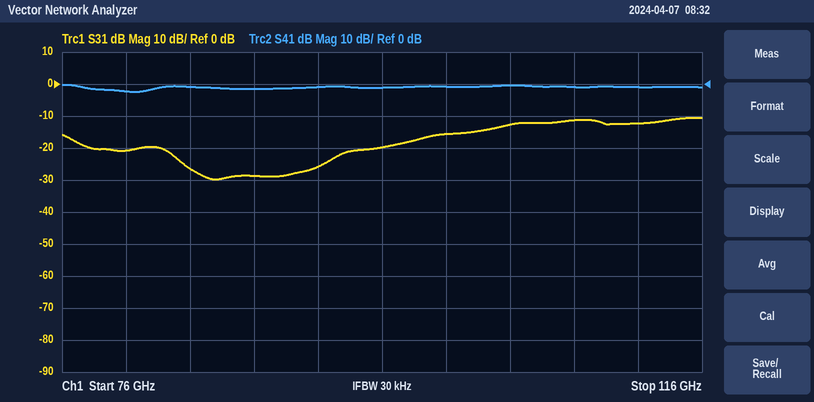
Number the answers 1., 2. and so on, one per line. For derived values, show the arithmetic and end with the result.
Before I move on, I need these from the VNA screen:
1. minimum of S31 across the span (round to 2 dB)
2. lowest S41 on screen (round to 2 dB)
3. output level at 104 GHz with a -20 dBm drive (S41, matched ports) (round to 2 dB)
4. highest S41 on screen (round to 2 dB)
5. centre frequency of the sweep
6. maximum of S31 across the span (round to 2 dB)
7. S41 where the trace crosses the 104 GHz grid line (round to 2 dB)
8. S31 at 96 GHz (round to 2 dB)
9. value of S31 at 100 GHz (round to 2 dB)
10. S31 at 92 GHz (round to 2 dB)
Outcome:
1. -30 dB
2. -2 dB
3. -20 dBm + (0 dB) = -20 dBm
4. 0 dB
5. 96 GHz
6. -10 dB
7. 0 dB
8. -20 dB
9. -16 dB
10. -26 dB
